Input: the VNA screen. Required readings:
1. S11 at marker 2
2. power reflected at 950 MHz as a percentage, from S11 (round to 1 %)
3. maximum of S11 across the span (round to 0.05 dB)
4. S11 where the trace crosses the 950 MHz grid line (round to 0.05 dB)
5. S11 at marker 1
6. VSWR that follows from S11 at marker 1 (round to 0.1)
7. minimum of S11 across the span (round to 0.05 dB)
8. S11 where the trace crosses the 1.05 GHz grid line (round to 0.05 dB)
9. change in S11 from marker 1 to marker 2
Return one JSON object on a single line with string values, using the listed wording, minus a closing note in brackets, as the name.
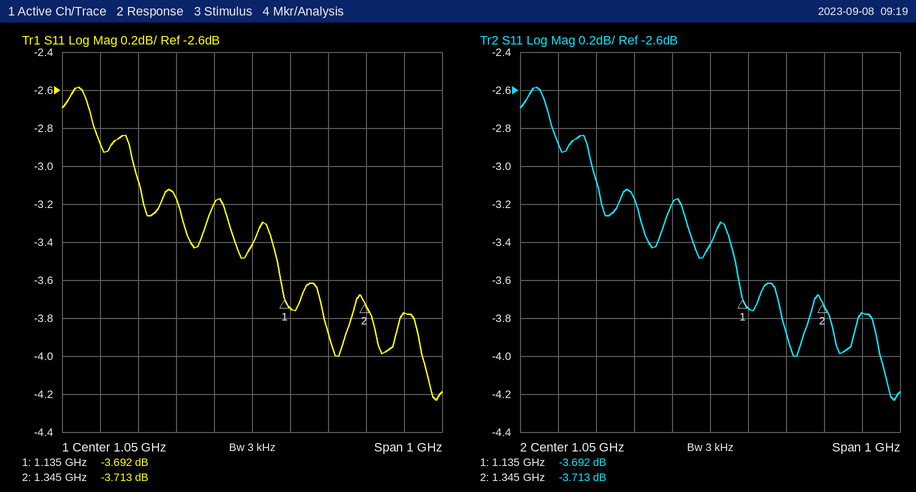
{"S11 at marker 2": "-3.713 dB", "power reflected at 950 MHz as a percentage, from S11": "48 %", "maximum of S11 across the span": "-2.60 dB", "S11 where the trace crosses the 950 MHz grid line": "-3.20 dB", "S11 at marker 1": "-3.692 dB", "VSWR that follows from S11 at marker 1": "4.8", "minimum of S11 across the span": "-4.25 dB", "S11 where the trace crosses the 1.05 GHz grid line": "-3.40 dB", "change in S11 from marker 1 to marker 2": "-0.021 dB"}
